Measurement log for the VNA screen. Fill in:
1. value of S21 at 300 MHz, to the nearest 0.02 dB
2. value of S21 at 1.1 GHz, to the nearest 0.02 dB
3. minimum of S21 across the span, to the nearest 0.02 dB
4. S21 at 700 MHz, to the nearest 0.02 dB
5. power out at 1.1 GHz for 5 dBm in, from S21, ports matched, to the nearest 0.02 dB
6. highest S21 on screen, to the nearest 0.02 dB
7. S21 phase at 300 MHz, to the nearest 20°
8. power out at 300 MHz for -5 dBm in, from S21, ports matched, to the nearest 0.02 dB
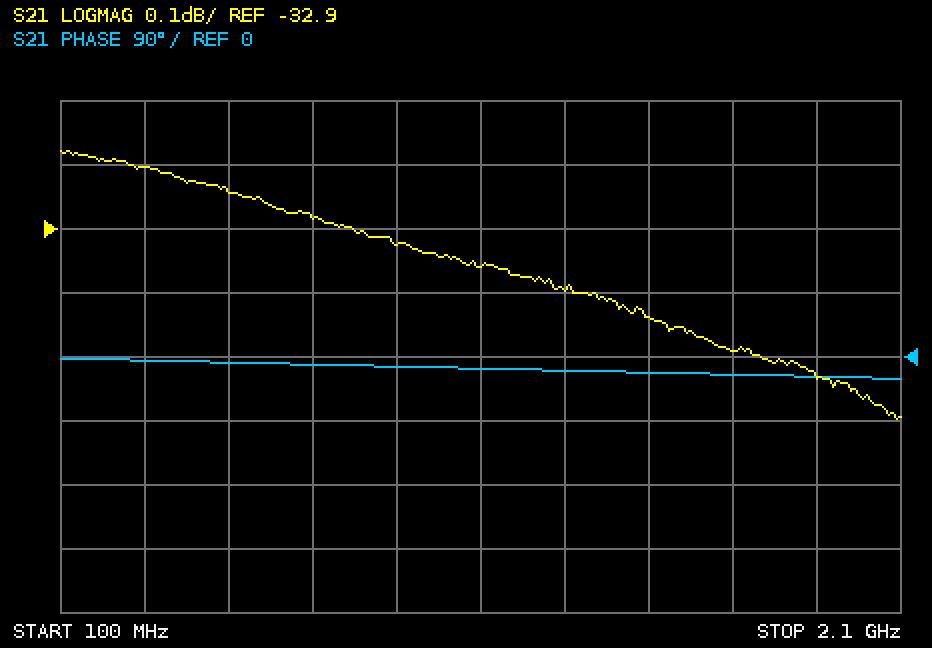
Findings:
-32.80 dB
-32.96 dB
-33.20 dB
-32.88 dB
-27.96 dBm
-32.78 dB
0°
-37.80 dBm
